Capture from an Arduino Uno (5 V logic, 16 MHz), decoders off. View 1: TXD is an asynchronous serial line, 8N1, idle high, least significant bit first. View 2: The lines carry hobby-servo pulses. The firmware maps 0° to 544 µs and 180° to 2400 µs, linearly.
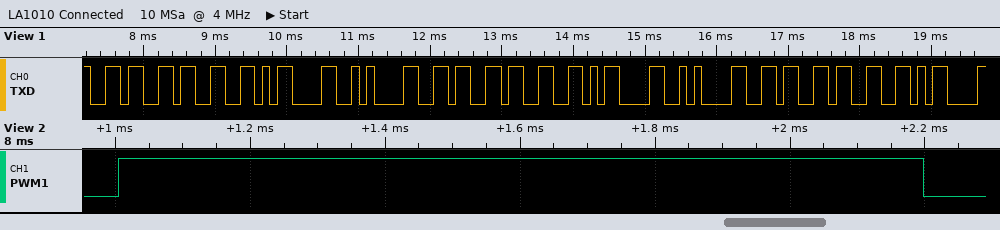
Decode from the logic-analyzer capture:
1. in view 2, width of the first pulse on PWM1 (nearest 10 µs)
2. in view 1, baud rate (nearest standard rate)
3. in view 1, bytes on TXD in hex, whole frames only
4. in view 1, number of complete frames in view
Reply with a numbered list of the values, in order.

1. 1190 µs
2. 9600 baud
3. 0x36 0x33 0x0D 0x0A 0x36 0x33 0x0D 0x0A 0x36 0x33 0x0D
4. 11
